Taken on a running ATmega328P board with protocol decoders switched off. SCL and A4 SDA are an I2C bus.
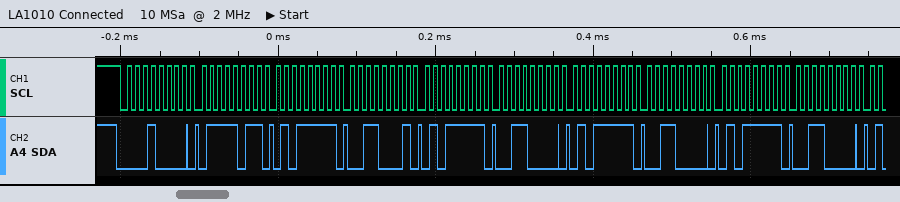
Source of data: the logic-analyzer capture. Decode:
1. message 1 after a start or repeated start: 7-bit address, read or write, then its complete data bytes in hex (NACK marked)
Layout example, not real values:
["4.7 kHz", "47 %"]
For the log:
["0x08 write: 7B 5F 31 5F 30 5F 30 5F 30"]
